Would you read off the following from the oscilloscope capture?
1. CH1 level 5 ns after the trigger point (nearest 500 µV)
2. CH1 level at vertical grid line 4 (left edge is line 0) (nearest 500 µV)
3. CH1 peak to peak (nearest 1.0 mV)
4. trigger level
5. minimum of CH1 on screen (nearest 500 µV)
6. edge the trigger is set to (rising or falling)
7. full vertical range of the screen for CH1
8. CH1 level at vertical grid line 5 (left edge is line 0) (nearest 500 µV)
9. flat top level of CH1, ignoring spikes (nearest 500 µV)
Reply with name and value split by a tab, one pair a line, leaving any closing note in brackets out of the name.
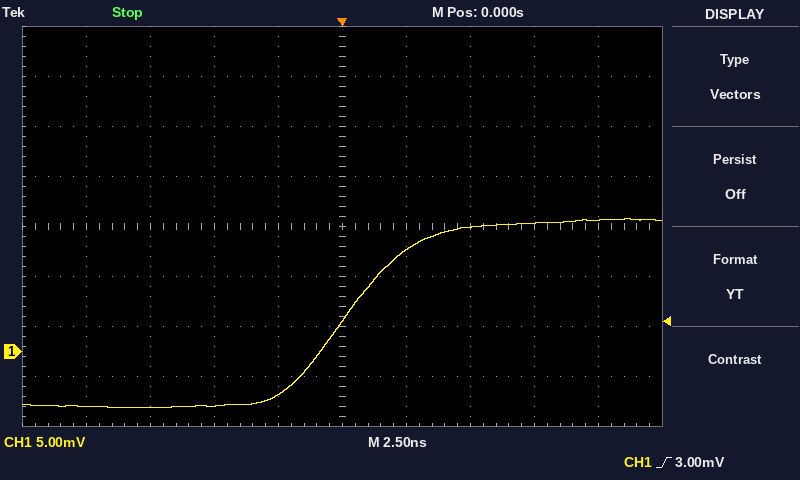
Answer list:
CH1 level 5 ns after the trigger point	12.5 mV
CH1 level at vertical grid line 4 (left edge is line 0)	-4.5 mV
CH1 peak to peak	19.0 mV
trigger level	3.00 mV
minimum of CH1 on screen	-5.5 mV
edge the trigger is set to	rising
full vertical range of the screen for CH1	40 mV
CH1 level at vertical grid line 5 (left edge is line 0)	3.0 mV
flat top level of CH1, ignoring spikes	13.0 mV
